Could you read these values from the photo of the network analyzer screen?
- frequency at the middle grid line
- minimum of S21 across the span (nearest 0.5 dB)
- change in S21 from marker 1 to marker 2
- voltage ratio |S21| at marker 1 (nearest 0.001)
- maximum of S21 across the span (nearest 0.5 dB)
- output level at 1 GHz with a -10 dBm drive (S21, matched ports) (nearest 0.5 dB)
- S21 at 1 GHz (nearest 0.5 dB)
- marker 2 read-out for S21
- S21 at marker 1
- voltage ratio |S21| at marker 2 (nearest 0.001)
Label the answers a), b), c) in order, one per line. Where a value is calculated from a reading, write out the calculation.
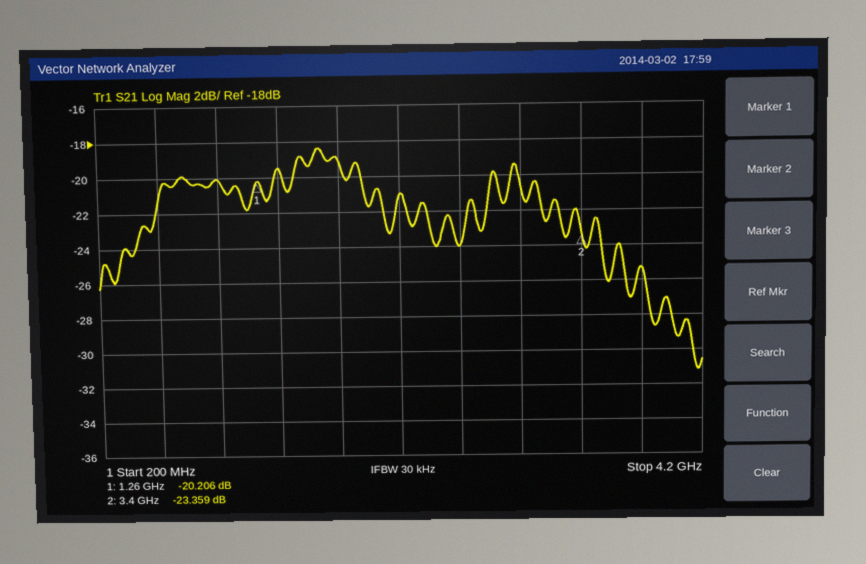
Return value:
a) 2.2 GHz
b) -31.0 dB
c) -23.359 − (-20.206) = -3.153 dB
d) 10^(-20.206/20) ≈ 0.098
e) -18.5 dB
f) -10 dBm + (-20.0 dB) = -30.0 dBm
g) -20.0 dB
h) -23.359 dB
i) -20.206 dB
j) 10^(-23.359/20) ≈ 0.068
